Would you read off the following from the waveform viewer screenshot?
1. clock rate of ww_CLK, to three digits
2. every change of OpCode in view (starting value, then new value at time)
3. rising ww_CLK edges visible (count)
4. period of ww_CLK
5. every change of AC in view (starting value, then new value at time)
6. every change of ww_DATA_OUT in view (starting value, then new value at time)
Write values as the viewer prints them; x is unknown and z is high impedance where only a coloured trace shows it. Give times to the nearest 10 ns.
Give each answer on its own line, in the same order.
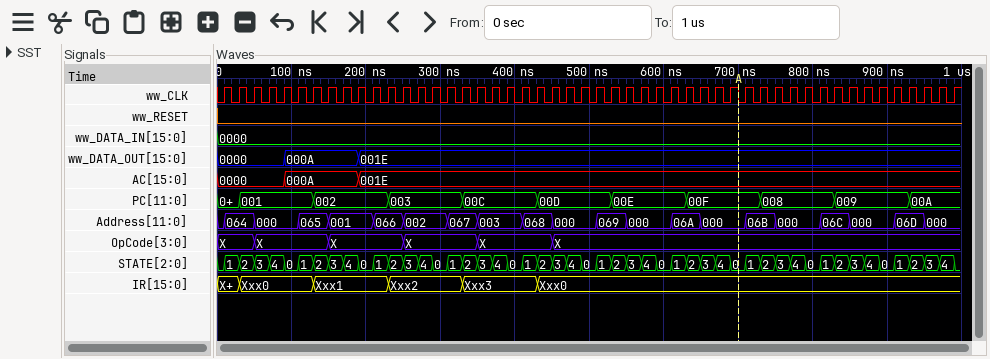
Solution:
50.0 MHz
X, X at 50 ns, X at 150 ns, X at 250 ns, X at 350 ns, X at 450 ns
50
20 ns
0000, 000A at 90 ns, 001E at 190 ns
0000, 000A at 90 ns, 001E at 190 ns
